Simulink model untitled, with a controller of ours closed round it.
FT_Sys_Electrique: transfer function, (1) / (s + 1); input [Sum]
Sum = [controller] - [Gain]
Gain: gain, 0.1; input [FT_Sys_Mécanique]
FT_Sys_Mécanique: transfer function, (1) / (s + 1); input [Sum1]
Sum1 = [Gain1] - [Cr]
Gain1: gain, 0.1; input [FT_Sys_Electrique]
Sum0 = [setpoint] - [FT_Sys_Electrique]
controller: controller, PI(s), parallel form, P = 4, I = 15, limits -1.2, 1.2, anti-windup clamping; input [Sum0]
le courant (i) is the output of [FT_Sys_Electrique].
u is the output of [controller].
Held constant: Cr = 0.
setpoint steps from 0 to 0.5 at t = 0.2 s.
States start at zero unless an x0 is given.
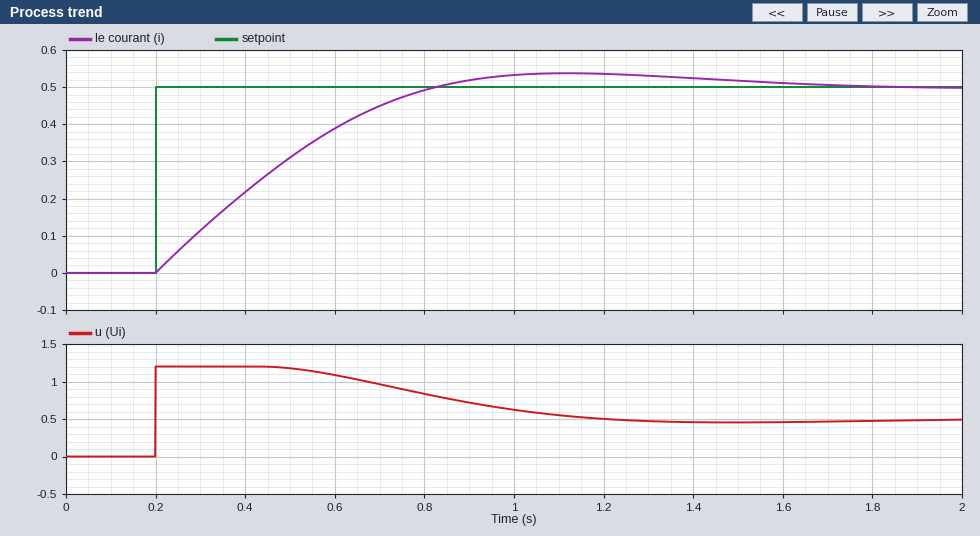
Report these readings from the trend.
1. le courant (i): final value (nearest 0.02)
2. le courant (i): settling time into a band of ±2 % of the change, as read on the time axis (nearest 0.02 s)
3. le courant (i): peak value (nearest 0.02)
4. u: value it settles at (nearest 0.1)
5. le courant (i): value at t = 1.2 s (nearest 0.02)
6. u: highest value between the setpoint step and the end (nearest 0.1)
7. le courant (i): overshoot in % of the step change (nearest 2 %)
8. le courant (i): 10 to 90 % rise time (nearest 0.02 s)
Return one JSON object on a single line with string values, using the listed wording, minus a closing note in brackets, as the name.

{"le courant (i): final value": "0.50", "le courant (i): settling time into a band of ±2 % of the change, as read on the time axis": "1.62 s", "le courant (i): peak value": "0.54", "u: value it settles at": "0.5", "le courant (i): value at t = 1.2 s": "0.54", "u: highest value between the setpoint step and the end": "1.2", "le courant (i): overshoot in % of the step change": "8 %", "le courant (i): 10 to 90 % rise time": "0.46 s"}
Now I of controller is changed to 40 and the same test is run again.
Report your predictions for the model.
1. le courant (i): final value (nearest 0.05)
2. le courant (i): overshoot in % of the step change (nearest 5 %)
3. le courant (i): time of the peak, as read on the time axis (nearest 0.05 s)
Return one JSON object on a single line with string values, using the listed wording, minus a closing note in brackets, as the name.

{"le courant (i): final value": "0.50", "le courant (i): overshoot in % of the step change": "10 %", "le courant (i): time of the peak, as read on the time axis": "0.95 s"}
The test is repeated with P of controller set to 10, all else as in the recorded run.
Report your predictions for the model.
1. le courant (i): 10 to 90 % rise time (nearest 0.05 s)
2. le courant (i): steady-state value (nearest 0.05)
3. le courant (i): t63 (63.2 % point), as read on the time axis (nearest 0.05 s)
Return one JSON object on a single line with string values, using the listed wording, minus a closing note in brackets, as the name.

{"le courant (i): 10 to 90 % rise time": "0.50 s", "le courant (i): steady-state value": "0.50", "le courant (i): t63 (63.2 % point), as read on the time axis": "0.50 s"}
